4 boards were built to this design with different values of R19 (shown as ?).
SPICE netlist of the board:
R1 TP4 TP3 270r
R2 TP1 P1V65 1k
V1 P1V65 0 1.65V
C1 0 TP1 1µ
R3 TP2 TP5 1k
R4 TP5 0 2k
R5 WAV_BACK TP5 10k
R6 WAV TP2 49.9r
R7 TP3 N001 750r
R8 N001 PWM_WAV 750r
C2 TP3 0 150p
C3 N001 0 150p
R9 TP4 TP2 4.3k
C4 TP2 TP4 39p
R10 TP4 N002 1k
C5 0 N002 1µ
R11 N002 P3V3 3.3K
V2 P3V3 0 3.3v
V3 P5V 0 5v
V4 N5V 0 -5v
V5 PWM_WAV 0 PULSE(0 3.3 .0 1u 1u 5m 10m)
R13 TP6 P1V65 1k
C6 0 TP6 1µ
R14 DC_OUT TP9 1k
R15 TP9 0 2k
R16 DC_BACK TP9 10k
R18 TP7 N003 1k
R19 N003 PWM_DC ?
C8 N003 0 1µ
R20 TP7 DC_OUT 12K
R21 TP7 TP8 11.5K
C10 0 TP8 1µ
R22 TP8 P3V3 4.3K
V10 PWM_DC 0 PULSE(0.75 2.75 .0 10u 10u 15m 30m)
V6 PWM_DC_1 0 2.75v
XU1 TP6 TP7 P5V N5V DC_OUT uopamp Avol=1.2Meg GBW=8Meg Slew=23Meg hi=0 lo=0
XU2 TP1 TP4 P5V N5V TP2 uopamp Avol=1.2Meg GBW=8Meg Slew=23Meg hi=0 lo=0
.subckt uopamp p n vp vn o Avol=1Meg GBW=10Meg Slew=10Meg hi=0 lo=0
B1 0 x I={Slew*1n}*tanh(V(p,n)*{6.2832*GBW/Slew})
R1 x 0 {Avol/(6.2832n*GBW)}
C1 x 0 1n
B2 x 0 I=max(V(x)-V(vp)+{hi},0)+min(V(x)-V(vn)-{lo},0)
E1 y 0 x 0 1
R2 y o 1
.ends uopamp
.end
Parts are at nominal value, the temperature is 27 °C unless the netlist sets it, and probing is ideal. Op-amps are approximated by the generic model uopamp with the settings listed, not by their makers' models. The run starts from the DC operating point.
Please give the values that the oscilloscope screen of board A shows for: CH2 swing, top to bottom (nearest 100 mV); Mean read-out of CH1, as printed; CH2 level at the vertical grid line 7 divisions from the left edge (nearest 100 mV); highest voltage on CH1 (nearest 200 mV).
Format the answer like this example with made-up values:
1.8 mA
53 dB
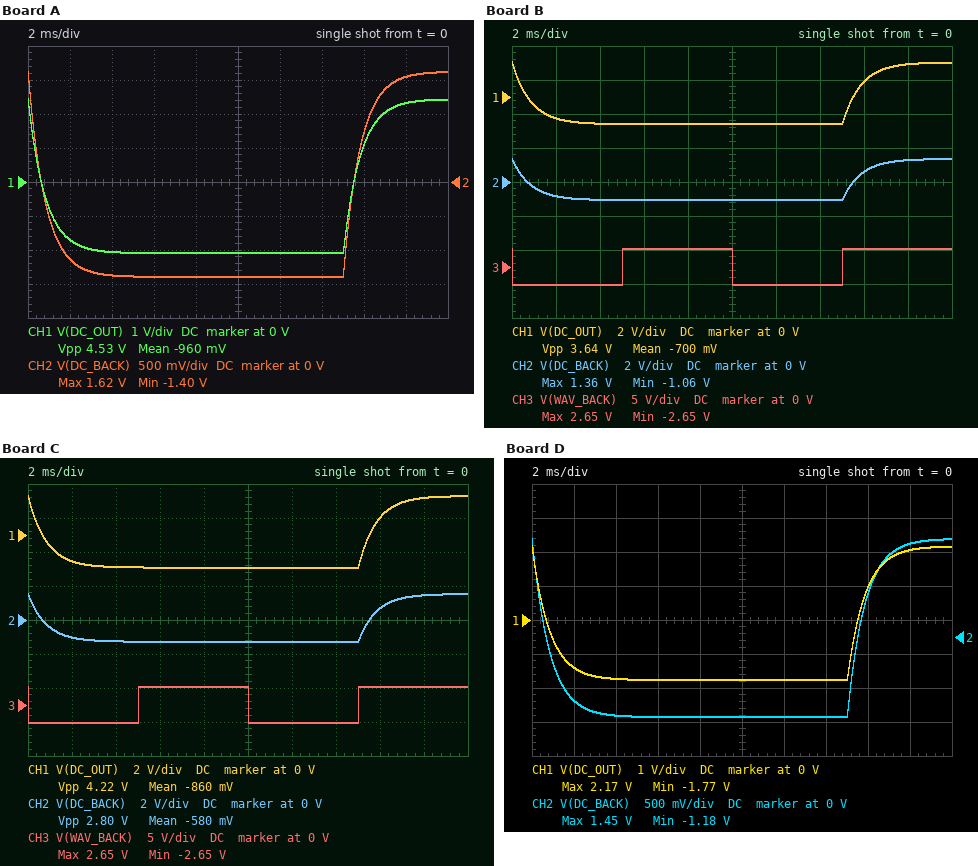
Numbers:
3.0 V
-960 mV
-1.4 V
2.4 V
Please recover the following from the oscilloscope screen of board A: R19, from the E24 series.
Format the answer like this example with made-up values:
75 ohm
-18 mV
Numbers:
4.3 kΩ
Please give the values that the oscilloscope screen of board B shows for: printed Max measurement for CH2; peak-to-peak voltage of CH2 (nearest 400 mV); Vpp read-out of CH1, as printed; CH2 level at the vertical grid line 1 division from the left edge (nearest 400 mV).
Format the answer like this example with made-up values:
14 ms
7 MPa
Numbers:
1.36 V
2.4 V
3.64 V
-800 mV
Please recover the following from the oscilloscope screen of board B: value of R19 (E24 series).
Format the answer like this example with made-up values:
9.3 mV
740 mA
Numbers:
5.6 kΩ
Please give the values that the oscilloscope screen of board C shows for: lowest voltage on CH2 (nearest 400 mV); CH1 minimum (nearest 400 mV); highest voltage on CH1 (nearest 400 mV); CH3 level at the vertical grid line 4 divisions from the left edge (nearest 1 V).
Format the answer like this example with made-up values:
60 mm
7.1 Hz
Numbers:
-1.2 V
-2.0 V
2.4 V
3 V
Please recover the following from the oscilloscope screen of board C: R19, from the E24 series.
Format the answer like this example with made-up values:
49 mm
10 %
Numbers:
4.7 kΩ
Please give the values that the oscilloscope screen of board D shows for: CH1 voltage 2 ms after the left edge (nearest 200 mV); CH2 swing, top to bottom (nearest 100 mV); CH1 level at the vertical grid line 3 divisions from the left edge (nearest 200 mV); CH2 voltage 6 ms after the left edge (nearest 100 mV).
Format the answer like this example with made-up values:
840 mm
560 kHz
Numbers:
-1.4 V
2.6 V
-1.8 V
-1.2 V
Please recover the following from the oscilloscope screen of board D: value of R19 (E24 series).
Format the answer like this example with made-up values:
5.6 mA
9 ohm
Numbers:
5.1 kΩ
